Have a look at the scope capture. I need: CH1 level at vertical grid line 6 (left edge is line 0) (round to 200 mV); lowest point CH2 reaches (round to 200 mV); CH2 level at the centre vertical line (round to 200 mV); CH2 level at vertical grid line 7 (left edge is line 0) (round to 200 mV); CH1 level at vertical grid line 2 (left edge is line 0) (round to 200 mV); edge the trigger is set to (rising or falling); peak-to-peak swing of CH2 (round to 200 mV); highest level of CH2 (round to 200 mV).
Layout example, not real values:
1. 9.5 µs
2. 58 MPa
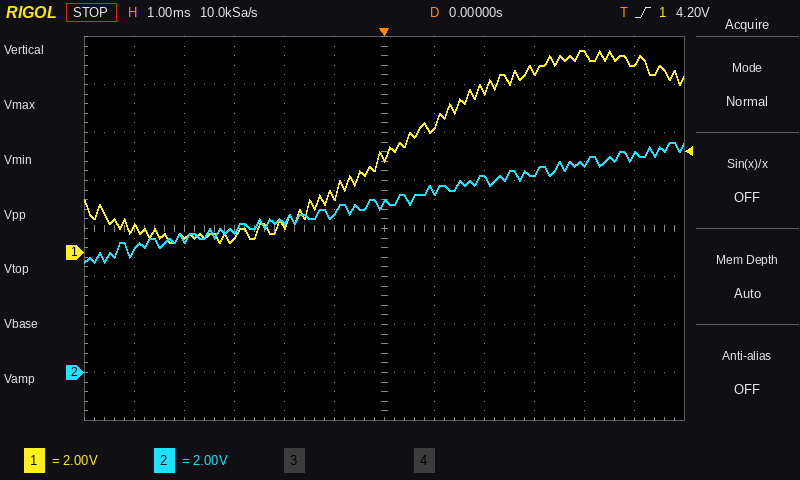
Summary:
1. 4.0 V
2. 4.6 V
3. 7.0 V
4. 7.6 V
5. 600 mV
6. rising
7. 5.0 V
8. 9.6 V
